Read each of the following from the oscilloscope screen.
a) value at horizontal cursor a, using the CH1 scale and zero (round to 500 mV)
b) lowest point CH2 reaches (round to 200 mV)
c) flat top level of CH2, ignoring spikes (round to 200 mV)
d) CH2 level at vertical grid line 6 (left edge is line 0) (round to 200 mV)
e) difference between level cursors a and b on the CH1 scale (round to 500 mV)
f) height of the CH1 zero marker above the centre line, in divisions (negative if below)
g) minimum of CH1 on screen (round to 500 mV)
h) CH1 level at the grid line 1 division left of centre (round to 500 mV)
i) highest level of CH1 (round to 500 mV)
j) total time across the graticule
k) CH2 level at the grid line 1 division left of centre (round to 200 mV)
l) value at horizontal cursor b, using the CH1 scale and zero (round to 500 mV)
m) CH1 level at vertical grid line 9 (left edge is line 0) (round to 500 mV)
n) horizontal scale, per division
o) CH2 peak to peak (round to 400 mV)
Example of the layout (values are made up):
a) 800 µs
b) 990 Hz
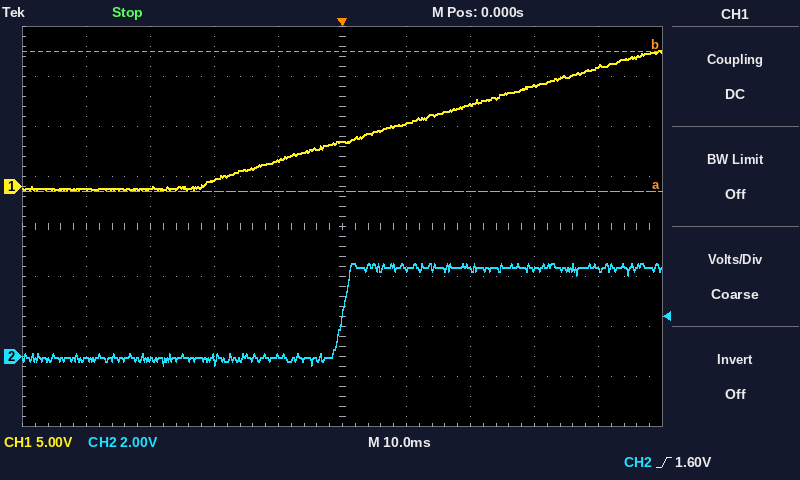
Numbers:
a) -500 mV
b) -400 mV
c) 3.6 V
d) 3.6 V
e) 14.0 V
f) +0.8 div
g) -500 mV
h) 2.5 V
i) 13.5 V
j) 100 ms
k) 0.0 V
l) 13.5 V
m) 12.0 V
n) 10 ms
o) 4.0 V
